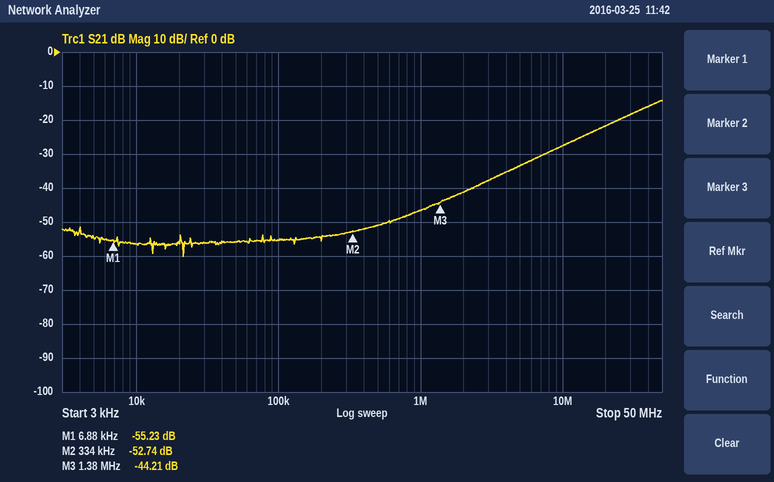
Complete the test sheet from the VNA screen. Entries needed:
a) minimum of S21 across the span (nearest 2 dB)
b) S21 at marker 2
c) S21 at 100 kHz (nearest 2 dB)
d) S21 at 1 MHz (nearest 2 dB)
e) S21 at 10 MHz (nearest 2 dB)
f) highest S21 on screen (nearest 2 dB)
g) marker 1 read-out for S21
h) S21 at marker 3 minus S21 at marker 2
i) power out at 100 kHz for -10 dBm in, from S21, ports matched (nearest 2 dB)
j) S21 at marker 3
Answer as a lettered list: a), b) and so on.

a) -60 dB
b) -52.74 dB
c) -56 dB
d) -46 dB
e) -28 dB
f) -14 dB
g) -55.23 dB
h) 8.53 dB
i) -66 dBm
j) -44.21 dB
